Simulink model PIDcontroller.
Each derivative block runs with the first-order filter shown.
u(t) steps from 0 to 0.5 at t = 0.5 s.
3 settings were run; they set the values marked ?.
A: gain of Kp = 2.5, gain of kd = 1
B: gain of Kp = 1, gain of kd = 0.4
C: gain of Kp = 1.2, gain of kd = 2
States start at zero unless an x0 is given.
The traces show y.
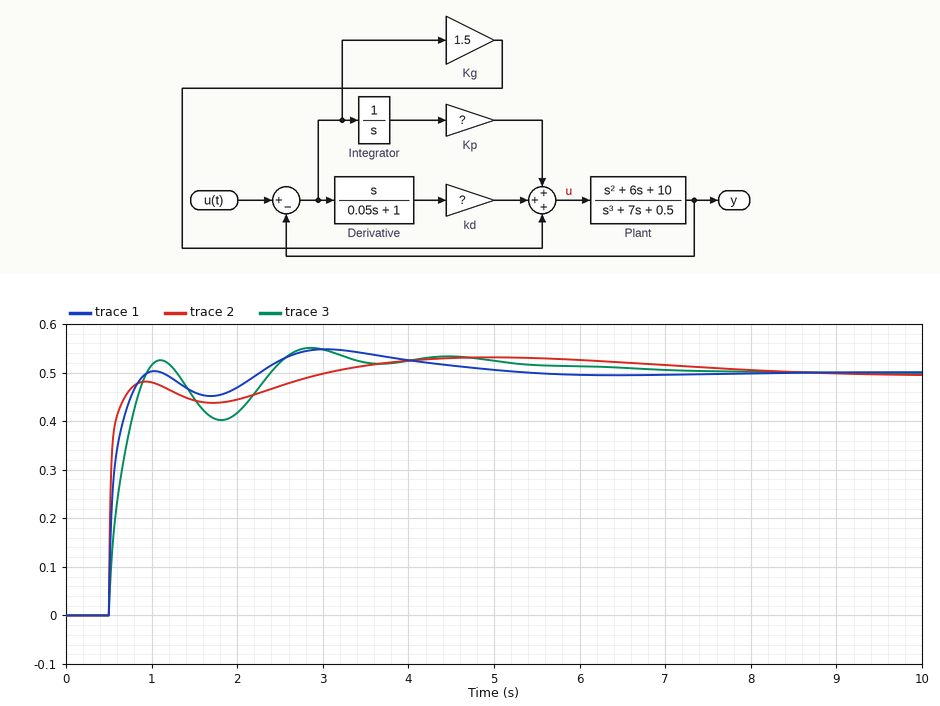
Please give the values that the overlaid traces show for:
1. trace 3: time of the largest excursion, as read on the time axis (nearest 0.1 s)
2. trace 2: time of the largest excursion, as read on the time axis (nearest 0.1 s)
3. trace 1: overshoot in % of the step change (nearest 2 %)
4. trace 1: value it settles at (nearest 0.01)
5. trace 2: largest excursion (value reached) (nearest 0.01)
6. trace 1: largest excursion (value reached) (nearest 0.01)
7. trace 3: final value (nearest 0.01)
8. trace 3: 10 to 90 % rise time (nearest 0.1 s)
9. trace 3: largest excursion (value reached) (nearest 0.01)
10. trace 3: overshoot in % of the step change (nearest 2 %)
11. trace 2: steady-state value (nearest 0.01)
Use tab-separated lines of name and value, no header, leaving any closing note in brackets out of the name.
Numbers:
trace 3: time of the largest excursion, as read on the time axis	2.9 s
trace 2: time of the largest excursion, as read on the time axis	5.0 s
trace 1: overshoot in % of the step change	10 %
trace 1: value it settles at	0.50
trace 2: largest excursion (value reached)	0.53
trace 1: largest excursion (value reached)	0.55
trace 3: final value	0.50
trace 3: 10 to 90 % rise time	0.3 s
trace 3: largest excursion (value reached)	0.55
trace 3: overshoot in % of the step change	10 %
trace 2: steady-state value	0.50
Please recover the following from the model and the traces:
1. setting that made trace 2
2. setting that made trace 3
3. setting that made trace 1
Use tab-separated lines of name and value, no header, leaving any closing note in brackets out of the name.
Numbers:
setting that made trace 2	C
setting that made trace 3	B
setting that made trace 1	A
